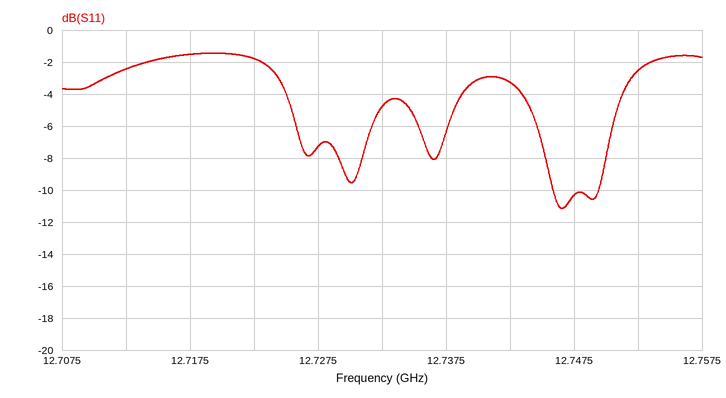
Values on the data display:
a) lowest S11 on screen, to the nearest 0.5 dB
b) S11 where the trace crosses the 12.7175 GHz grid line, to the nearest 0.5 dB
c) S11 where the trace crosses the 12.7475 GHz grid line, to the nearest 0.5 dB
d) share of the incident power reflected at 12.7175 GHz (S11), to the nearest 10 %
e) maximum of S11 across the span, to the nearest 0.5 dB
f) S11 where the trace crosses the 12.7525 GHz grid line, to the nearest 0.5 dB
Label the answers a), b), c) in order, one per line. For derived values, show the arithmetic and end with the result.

a) -11.0 dB
b) -1.5 dB
c) -10.5 dB
d) 10^(-1.5/10) ≈ 70.8 %, so 70 % to the nearest 10 %
e) -1.5 dB
f) -2.5 dB
